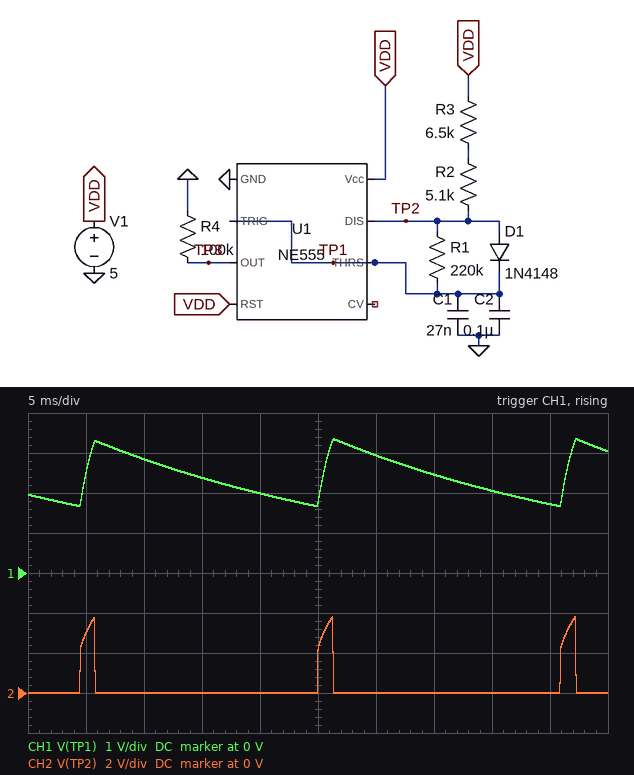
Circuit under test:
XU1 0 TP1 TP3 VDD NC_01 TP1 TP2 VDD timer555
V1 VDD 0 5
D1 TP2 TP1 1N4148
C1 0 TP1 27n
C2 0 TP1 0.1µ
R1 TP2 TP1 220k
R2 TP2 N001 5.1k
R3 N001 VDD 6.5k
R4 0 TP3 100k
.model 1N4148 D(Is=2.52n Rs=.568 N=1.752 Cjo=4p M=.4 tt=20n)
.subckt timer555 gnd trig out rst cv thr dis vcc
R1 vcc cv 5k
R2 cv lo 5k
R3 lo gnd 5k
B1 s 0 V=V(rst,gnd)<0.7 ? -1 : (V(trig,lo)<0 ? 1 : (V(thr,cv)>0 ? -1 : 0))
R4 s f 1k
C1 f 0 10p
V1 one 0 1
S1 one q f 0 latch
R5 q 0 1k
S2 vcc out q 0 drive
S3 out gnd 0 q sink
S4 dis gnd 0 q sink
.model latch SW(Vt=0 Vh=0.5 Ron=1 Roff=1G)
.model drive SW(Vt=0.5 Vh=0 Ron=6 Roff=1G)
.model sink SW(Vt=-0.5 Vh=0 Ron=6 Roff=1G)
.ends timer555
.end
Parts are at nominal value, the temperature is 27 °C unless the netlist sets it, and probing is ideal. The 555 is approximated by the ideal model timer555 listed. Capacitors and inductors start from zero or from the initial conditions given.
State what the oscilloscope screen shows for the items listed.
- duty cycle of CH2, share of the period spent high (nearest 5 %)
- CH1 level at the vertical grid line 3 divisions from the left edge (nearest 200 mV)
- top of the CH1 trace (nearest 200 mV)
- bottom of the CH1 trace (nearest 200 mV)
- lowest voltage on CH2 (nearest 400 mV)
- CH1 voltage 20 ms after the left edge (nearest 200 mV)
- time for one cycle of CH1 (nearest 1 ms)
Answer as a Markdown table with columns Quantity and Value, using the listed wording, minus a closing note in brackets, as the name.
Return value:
| Quantity | Value |
|---|---|
| duty cycle of CH2, share of the period spent high | 5 % |
| CH1 level at the vertical grid line 3 divisions from the left edge | 2.4 V |
| top of the CH1 trace | 3.4 V |
| bottom of the CH1 trace | 1.6 V |
| lowest voltage on CH2 | 0 V |
| CH1 voltage 20 ms after the left edge | 2.0 V |
| time for one cycle of CH1 | 21 ms |
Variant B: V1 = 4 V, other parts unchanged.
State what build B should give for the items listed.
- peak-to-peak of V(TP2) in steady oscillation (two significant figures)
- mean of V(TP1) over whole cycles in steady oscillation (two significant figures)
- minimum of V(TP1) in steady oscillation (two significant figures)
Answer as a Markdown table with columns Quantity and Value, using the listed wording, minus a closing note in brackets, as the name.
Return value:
| Quantity | Value |
|---|---|
| peak-to-peak of V(TP2) in steady oscillation | 3.1 V |
| mean of V(TP1) over whole cycles in steady oscillation | 1.9 V |
| minimum of V(TP1) in steady oscillation | 1.3 V |
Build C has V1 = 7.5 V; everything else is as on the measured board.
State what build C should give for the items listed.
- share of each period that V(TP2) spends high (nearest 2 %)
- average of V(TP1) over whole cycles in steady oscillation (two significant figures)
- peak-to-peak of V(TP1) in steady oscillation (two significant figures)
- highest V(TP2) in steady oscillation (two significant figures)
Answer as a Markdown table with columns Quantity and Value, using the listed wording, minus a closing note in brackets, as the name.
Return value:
| Quantity | Value |
|---|---|
| share of each period that V(TP2) spends high | 6 % |
| average of V(TP1) over whole cycles in steady oscillation | 3.6 V |
| peak-to-peak of V(TP1) in steady oscillation | 2.5 V |
| highest V(TP2) in steady oscillation | 5.5 V |
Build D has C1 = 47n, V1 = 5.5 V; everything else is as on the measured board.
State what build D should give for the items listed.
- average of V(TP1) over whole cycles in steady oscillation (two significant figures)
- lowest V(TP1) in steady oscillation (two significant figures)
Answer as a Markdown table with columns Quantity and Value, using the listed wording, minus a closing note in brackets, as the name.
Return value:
| Quantity | Value |
|---|---|
| average of V(TP1) over whole cycles in steady oscillation | 2.7 V |
| lowest V(TP1) in steady oscillation | 1.8 V |
